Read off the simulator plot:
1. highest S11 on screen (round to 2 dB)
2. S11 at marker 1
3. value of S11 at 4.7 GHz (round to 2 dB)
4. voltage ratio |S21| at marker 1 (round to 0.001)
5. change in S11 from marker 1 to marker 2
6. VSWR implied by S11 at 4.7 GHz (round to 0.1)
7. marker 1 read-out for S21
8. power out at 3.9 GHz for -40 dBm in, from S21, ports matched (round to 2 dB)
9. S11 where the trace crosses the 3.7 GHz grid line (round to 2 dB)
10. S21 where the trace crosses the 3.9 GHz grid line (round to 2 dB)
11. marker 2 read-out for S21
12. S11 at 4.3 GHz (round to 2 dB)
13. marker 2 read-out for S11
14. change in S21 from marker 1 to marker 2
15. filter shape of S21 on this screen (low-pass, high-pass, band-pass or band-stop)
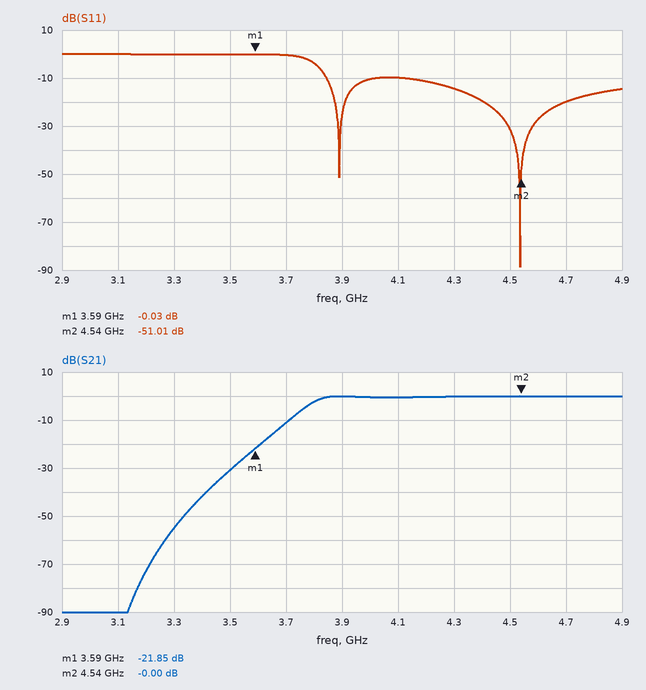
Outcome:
0 dB
-0.03 dB
-20 dB
0.081
-50.98 dB
1.2
-21.85 dB
-40 dBm
0 dB
0 dB
-0.00 dB
-14 dB
-51.01 dB
21.85 dB
high-pass
